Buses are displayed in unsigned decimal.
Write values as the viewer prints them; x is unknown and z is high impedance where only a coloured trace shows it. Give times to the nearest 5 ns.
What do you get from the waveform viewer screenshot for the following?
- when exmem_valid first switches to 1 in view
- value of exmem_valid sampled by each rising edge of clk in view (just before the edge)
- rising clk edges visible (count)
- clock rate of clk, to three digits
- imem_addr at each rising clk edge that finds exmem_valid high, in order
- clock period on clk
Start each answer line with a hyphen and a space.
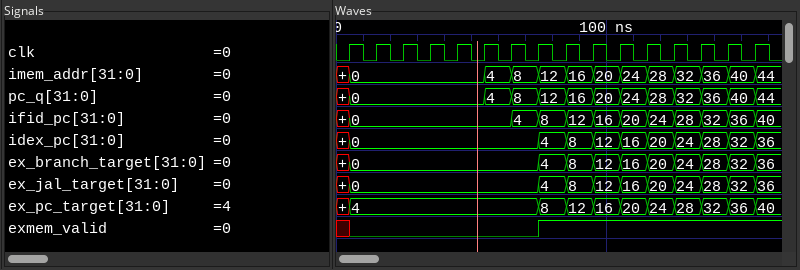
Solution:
- 75 ns
- x 0 0 0 0 0 0 0 1 1 1 1 1 1 1 1
- 16
- 100 MHz
- 12, 16, 20, 24, 28, 32, 36, 40
- 10 ns
